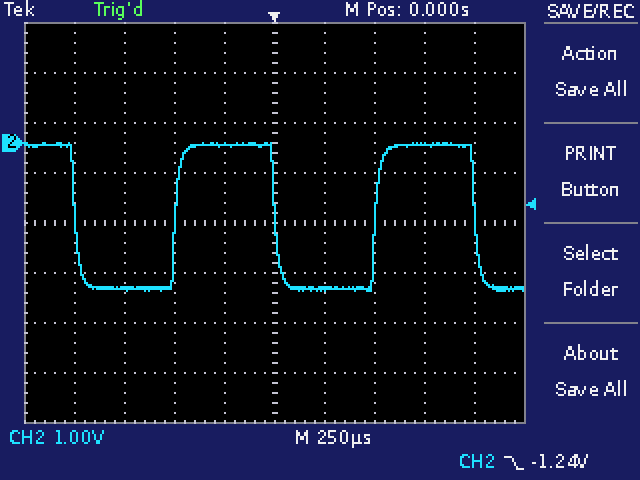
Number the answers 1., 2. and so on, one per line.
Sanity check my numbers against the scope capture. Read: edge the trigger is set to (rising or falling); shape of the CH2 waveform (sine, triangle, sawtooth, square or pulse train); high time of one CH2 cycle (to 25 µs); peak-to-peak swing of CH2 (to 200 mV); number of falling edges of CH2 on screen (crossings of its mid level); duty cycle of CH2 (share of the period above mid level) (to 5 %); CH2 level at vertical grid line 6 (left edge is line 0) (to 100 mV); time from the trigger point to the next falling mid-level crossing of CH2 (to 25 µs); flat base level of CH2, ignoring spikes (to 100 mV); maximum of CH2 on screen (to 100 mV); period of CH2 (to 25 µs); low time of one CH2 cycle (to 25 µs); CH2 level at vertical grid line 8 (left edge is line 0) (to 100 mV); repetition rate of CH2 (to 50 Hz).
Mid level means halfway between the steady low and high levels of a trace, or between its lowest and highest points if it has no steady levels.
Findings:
1. falling
2. square
3. 500 µs
4. 3.0 V
5. 3
6. 50 %
7. -2.9 V
8. 1.000 ms
9. -2.9 V
10. 0.0 V
11. 1.000 ms
12. 500 µs
13. 0.0 V
14. 1.00 kHz
